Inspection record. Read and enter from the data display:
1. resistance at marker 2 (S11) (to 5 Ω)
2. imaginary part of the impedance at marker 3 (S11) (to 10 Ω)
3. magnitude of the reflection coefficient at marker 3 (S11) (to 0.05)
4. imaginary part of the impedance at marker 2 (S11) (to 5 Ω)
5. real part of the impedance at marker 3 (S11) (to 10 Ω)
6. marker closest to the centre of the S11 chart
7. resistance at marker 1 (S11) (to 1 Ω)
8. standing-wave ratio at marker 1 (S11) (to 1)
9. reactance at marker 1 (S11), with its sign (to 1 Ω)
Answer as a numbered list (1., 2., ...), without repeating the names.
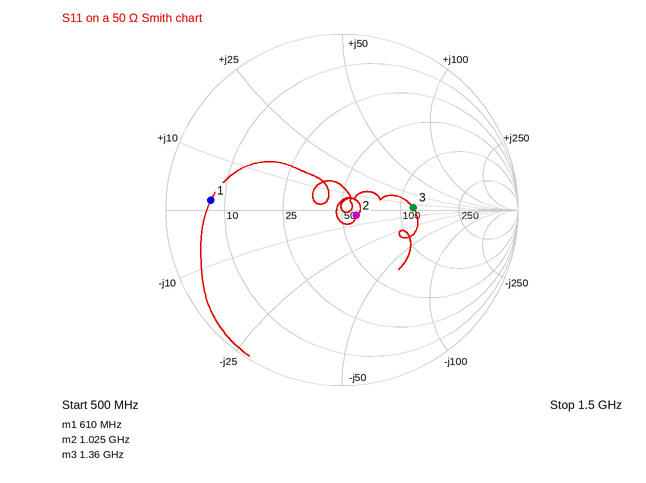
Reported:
1. 60 Ω
2. 0 Ω
3. 0.40
4. -5 Ω
5. 120 Ω
6. marker 2
7. 7 Ω
8. 7
9. +2 Ω
